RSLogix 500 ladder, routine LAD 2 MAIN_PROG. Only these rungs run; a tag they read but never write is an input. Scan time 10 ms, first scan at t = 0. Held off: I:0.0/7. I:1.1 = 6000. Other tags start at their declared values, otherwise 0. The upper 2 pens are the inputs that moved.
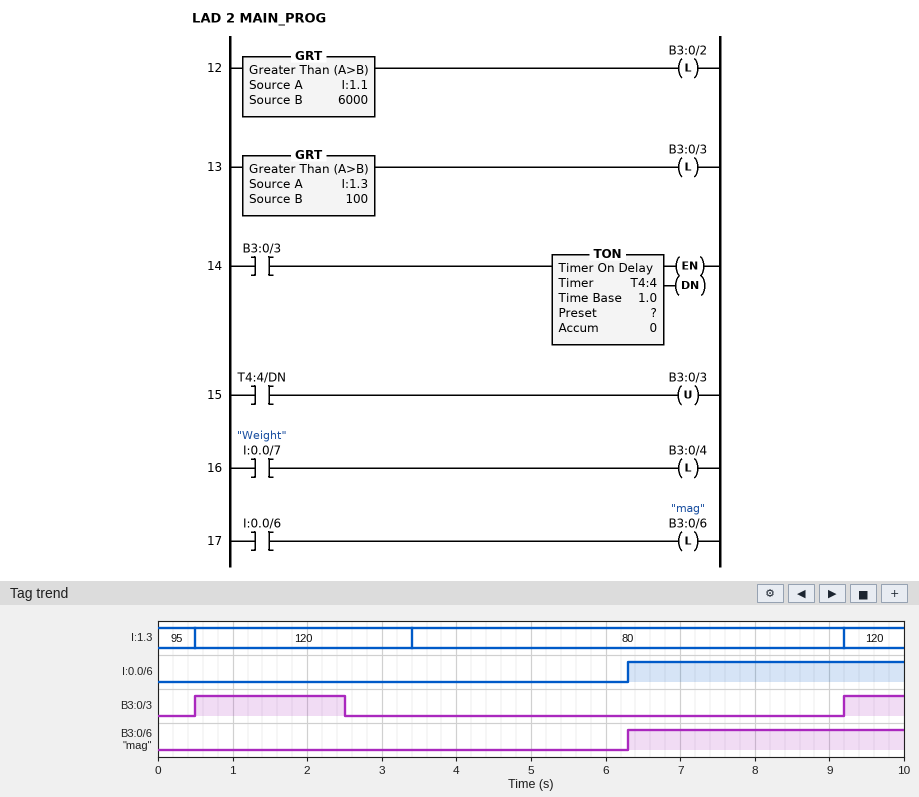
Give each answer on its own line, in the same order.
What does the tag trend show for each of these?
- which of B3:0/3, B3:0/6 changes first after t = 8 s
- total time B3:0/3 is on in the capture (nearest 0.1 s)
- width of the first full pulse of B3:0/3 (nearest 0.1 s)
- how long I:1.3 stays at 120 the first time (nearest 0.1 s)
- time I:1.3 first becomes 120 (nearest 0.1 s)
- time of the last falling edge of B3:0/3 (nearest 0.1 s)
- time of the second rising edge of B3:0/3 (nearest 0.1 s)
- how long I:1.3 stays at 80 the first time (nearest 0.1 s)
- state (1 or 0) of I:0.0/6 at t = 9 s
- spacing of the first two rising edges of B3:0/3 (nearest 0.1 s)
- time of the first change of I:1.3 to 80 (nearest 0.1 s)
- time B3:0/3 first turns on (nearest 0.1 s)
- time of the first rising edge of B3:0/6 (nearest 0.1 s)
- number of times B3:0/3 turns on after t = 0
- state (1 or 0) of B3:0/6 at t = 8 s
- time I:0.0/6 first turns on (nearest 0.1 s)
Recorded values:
B3:0/3
2.8 s
2.0 s
2.9 s
0.5 s
2.5 s
9.2 s
5.8 s
1
8.7 s
3.4 s
0.5 s
6.3 s
2
1
6.3 s
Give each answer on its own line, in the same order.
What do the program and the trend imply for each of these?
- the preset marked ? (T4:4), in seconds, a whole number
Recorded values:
2 s
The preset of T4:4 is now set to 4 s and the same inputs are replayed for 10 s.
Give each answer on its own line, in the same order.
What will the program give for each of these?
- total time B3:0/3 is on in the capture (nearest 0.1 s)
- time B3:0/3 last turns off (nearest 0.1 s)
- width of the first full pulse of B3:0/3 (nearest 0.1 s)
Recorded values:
4.8 s
4.5 s
4.0 s
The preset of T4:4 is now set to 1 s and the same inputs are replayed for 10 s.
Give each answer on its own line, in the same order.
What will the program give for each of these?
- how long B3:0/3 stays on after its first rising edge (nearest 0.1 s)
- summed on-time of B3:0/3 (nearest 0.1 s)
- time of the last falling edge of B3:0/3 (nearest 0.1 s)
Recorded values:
1.0 s
1.8 s
1.5 s
